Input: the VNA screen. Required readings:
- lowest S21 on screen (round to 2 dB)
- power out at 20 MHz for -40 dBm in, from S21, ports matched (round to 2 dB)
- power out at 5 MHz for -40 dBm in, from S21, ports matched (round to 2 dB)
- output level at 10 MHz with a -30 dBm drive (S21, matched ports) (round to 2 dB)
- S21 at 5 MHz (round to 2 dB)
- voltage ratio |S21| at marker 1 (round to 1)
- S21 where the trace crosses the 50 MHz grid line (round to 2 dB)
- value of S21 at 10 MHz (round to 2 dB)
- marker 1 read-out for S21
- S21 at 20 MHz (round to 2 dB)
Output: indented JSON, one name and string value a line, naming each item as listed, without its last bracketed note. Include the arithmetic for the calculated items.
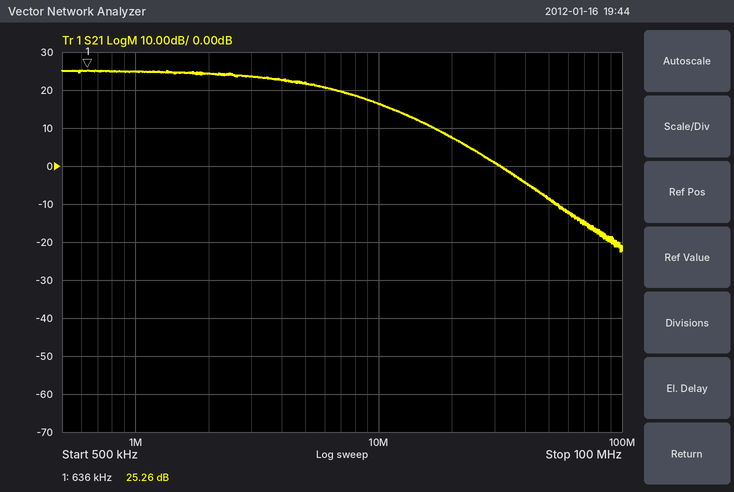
{
  "lowest S21 on screen": "-22 dB",
  "power out at 20 MHz for -40 dBm in, from S21, ports matched": "-40 dBm + (8 dB) = -32 dBm",
  "power out at 5 MHz for -40 dBm in, from S21, ports matched": "-40 dBm + (22 dB) = -18 dBm",
  "output level at 10 MHz with a -30 dBm drive (S21, matched ports)": "-30 dBm + (16 dB) = -14 dBm",
  "S21 at 5 MHz": "22 dB",
  "voltage ratio |S21| at marker 1": "10^(25.26/20) ≈ 18",
  "S21 where the trace crosses the 50 MHz grid line": "-8 dB",
  "value of S21 at 10 MHz": "16 dB",
  "marker 1 read-out for S21": "25.26 dB",
  "S21 at 20 MHz": "8 dB"
}
